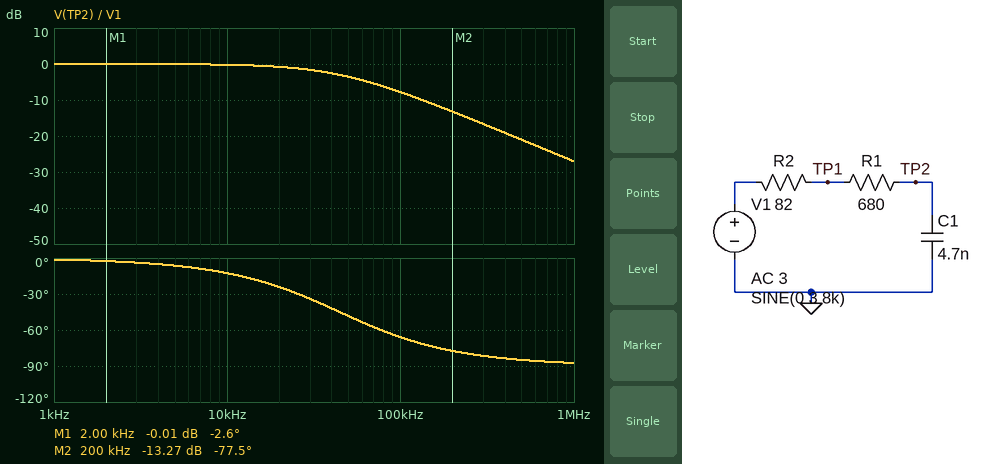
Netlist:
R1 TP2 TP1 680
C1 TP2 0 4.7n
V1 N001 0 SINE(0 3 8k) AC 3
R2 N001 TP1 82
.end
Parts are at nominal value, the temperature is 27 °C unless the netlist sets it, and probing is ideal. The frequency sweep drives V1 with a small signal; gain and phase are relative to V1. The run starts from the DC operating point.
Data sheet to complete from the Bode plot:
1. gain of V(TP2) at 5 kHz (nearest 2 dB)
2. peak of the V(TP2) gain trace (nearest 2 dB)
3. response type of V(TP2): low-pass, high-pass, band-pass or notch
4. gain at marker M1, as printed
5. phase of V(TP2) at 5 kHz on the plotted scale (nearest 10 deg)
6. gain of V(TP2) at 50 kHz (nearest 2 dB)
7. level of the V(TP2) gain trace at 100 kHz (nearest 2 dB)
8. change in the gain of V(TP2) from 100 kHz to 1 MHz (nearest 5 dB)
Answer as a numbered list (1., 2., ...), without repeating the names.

1. 0 dB
2. 0 dB
3. low-pass
4. -0.01 dB
5. -10 deg
6. -4 dB
7. -8 dB
8. -20 dB
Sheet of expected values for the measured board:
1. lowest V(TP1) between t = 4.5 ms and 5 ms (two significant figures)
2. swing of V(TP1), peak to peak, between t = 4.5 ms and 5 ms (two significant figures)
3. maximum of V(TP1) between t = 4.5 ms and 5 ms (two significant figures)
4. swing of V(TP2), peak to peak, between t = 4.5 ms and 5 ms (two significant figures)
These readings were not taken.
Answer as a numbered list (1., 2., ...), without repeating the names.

1. -3.0 V
2. 6.0 V
3. 3.0 V
4. 5.9 V
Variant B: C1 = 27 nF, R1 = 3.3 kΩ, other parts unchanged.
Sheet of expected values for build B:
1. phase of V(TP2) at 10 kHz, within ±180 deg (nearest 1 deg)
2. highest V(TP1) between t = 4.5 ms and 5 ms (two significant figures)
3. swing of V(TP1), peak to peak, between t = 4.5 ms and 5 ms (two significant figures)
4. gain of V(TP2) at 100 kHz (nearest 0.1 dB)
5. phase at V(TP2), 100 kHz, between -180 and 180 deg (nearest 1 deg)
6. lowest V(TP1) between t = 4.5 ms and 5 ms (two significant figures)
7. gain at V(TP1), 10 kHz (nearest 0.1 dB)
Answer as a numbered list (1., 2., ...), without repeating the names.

1. -80 deg
2. 2.9 V
3. 5.9 V
4. -35.2 dB
5. -89 deg
6. -2.9 V
7. -0.2 dB
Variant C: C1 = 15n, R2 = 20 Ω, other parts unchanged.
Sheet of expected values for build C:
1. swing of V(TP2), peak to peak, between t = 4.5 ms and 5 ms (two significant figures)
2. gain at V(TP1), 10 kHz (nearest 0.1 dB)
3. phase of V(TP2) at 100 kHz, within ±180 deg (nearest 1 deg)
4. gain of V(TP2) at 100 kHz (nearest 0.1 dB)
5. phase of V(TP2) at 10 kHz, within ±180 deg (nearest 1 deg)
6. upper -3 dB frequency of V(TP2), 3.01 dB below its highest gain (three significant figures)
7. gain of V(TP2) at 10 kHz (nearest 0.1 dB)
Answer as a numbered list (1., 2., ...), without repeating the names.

1. 5.3 V
2. -0.1 dB
3. -81 deg
4. -16.5 dB
5. -33 deg
6. 15.2 kHz
7. -1.6 dB
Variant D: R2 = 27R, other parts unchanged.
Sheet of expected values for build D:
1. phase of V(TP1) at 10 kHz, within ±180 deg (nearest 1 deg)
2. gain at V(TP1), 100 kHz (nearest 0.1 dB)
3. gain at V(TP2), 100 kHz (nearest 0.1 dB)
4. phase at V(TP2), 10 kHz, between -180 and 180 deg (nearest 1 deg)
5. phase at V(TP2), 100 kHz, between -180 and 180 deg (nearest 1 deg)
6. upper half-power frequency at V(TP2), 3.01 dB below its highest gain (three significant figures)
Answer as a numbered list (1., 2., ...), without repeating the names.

1. 0 deg
2. -0.3 dB
3. -7.3 dB
4. -12 deg
5. -64 deg
6. 47.9 kHz
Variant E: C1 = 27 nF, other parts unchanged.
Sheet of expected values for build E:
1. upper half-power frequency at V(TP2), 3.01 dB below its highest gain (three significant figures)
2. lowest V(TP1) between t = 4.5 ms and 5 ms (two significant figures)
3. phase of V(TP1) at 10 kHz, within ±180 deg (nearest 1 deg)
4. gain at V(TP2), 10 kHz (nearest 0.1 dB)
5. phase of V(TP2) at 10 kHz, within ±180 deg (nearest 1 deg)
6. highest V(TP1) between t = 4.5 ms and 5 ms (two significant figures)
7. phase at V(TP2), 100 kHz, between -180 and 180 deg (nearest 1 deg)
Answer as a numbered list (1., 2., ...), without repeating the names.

1. 7.74 kHz
2. -2.8 V
3. -3 deg
4. -4.3 dB
5. -52 deg
6. 2.8 V
7. -86 deg
